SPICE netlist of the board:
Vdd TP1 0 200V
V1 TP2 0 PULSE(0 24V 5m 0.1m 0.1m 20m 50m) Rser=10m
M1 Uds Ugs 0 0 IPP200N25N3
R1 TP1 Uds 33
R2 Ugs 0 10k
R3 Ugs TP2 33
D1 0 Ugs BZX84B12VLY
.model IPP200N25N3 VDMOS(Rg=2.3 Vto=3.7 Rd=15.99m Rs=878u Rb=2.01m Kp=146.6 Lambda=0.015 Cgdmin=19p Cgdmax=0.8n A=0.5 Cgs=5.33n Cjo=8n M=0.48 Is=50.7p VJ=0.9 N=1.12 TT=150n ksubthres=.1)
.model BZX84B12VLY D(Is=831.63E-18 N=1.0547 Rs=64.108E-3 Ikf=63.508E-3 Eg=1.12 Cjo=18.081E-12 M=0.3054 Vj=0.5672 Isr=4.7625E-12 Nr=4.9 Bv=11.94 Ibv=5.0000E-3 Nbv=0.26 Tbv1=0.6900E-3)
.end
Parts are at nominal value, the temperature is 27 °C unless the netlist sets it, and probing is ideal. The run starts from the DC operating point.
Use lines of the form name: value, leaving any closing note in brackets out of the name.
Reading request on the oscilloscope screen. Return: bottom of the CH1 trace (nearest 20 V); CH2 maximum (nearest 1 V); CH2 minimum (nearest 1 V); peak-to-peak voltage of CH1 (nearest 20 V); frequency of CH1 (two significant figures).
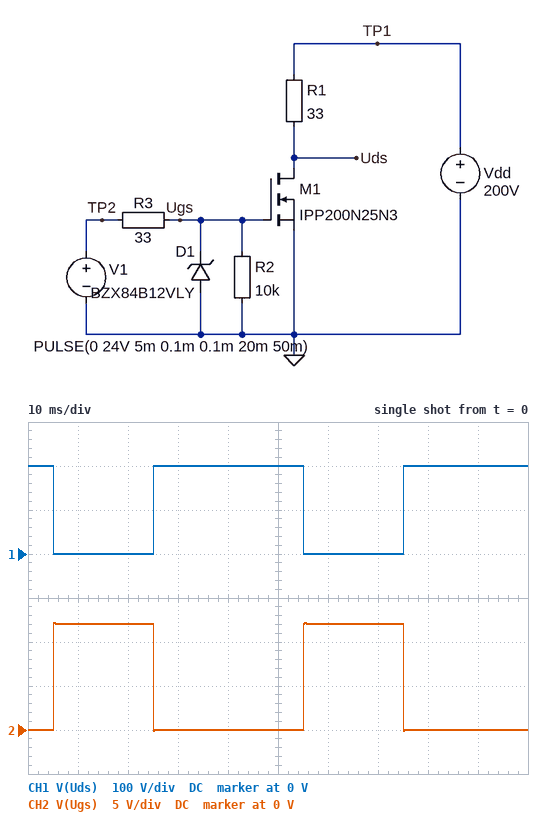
bottom of the CH1 trace: 0 V
CH2 maximum: 12 V
CH2 minimum: 0 V
peak-to-peak voltage of CH1: 200 V
frequency of CH1: 20 Hz
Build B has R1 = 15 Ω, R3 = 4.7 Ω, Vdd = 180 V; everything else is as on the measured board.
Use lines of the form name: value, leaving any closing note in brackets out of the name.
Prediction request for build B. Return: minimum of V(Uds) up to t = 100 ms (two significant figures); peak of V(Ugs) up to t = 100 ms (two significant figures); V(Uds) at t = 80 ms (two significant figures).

minimum of V(Uds) up to t = 100 ms: 210 mV
peak of V(Ugs) up to t = 100 ms: 12 V
V(Uds) at t = 80 ms: 180 V
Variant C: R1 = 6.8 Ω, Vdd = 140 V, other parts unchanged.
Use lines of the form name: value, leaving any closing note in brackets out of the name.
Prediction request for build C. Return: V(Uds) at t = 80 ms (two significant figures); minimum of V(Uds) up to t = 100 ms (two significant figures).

V(Uds) at t = 80 ms: 140 V
minimum of V(Uds) up to t = 100 ms: 360 mV
